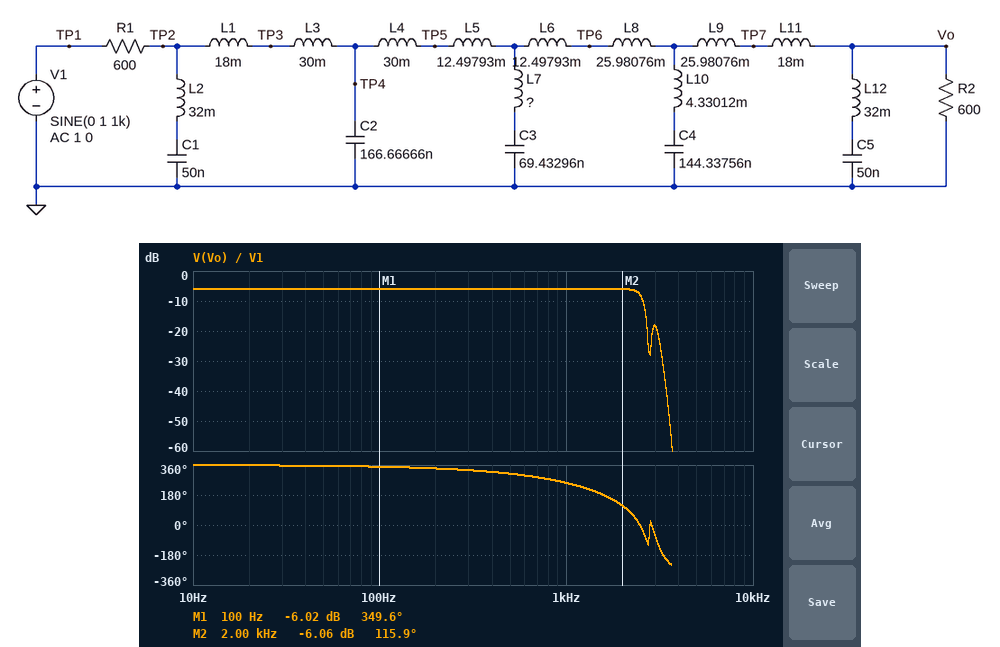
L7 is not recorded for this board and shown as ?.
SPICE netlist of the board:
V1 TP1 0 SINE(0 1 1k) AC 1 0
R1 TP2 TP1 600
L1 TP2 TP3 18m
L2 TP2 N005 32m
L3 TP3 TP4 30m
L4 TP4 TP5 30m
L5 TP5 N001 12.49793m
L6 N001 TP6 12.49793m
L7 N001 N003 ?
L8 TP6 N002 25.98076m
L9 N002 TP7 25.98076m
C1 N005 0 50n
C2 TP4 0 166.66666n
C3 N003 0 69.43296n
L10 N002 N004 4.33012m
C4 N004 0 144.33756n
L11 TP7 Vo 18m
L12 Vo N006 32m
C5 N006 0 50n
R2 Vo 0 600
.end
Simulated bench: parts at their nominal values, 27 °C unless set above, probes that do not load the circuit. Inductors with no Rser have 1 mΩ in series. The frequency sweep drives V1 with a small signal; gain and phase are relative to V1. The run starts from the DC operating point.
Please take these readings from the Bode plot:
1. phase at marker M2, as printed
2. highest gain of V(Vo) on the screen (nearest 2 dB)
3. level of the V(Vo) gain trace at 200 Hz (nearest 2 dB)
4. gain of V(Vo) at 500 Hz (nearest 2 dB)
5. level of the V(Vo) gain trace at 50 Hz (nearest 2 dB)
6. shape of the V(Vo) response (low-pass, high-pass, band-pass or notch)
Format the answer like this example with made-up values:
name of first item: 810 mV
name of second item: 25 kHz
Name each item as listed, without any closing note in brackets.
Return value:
phase at marker M2, as printed: 115.9 deg
highest gain of V(Vo) on the screen: -6 dB
level of the V(Vo) gain trace at 200 Hz: -6 dB
gain of V(Vo) at 500 Hz: -6 dB
level of the V(Vo) gain trace at 50 Hz: -6 dB
shape of the V(Vo) response: low-pass
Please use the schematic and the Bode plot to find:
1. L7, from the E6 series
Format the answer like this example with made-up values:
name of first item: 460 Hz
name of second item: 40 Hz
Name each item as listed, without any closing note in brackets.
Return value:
L7, from the E6 series: 47 mH
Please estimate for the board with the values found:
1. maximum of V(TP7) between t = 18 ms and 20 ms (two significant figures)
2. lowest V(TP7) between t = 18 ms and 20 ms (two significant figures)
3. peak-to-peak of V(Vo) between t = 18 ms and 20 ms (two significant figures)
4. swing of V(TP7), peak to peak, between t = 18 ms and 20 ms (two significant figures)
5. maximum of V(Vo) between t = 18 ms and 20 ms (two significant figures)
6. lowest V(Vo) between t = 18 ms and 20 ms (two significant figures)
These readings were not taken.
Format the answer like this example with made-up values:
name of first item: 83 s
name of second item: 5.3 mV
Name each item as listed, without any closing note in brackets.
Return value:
maximum of V(TP7) between t = 18 ms and 20 ms: 490 mV
lowest V(TP7) between t = 18 ms and 20 ms: -490 mV
peak-to-peak of V(Vo) between t = 18 ms and 20 ms: 1.0 V
swing of V(TP7), peak to peak, between t = 18 ms and 20 ms: 980 mV
maximum of V(Vo) between t = 18 ms and 20 ms: 500 mV
lowest V(Vo) between t = 18 ms and 20 ms: -500 mV
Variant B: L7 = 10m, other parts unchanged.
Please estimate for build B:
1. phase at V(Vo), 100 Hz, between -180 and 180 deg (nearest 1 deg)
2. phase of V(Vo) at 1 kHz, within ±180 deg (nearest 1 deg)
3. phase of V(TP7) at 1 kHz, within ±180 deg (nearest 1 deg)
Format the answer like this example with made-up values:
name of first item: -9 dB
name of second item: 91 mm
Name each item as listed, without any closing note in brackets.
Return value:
phase at V(Vo), 100 Hz, between -180 and 180 deg: -10 deg
phase of V(Vo) at 1 kHz, within ±180 deg: -106 deg
phase of V(TP7) at 1 kHz, within ±180 deg: -95 deg
